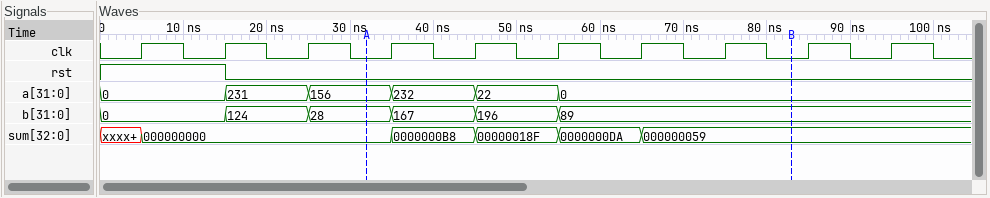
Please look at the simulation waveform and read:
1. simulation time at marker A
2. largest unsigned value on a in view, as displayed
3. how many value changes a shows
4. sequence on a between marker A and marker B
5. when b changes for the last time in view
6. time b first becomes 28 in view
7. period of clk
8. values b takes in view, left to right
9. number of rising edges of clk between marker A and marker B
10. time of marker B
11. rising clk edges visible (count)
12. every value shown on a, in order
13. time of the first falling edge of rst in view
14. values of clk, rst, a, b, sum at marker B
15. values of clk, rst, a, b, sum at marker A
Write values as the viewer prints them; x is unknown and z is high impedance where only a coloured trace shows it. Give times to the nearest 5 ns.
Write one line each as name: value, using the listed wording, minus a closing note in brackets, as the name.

simulation time at marker A: 30 ns
largest unsigned value on a in view, as displayed: 232
how many value changes a shows: 5
sequence on a between marker A and marker B: 156, 232, 22, 0
when b changes for the last time in view: 55 ns
time b first becomes 28 in view: 25 ns
period of clk: 10 ns
values b takes in view, left to right: 0, 124, 28, 167, 196, 89
number of rising edges of clk between marker A and marker B: 5
time of marker B: 85 ns
rising clk edges visible: 10
every value shown on a, in order: 0, 231, 156, 232, 22, 0
time of the first falling edge of rst in view: 15 ns
values of clk, rst, a, b, sum at marker B: clk=0, rst=0, a=0, b=89, sum=000000059
values of clk, rst, a, b, sum at marker A: clk=0, rst=0, a=156, b=28, sum=000000000
